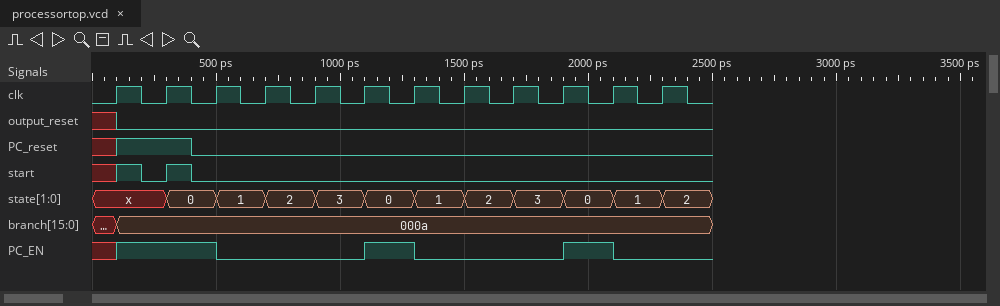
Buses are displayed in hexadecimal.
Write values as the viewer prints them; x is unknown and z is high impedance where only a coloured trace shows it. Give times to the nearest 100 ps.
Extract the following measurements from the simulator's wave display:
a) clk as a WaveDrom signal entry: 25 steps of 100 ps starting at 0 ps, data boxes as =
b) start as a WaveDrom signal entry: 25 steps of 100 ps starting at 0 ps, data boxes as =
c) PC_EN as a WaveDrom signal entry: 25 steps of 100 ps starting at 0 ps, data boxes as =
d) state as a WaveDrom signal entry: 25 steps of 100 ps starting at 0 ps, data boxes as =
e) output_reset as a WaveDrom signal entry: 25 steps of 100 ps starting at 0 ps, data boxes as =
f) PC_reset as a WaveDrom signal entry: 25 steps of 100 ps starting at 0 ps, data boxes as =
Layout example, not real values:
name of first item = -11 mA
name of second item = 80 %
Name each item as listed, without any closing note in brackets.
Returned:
clk as a WaveDrom signal entry: 25 steps of 100 ps starting at 0 ps, data boxes as = = {name: 'clk', wave: '0101010101010101010101010'}
start as a WaveDrom signal entry: 25 steps of 100 ps starting at 0 ps, data boxes as = = {name: 'start', wave: 'x1010....................'}
PC_EN as a WaveDrom signal entry: 25 steps of 100 ps starting at 0 ps, data boxes as = = {name: 'PC_EN', wave: 'x1...0.....1.0.....1.0...'}
state as a WaveDrom signal entry: 25 steps of 100 ps starting at 0 ps, data boxes as = = {name: 'state', wave: 'x..=.=.=.=.=.=.=.=.=.=.=.', data: '0 1 2 3 0 1 2 3 0 1 2'}
output_reset as a WaveDrom signal entry: 25 steps of 100 ps starting at 0 ps, data boxes as = = {name: 'output_reset', wave: 'x0.......................'}
PC_reset as a WaveDrom signal entry: 25 steps of 100 ps starting at 0 ps, data boxes as = = {name: 'PC_reset', wave: 'x1..0....................'}
